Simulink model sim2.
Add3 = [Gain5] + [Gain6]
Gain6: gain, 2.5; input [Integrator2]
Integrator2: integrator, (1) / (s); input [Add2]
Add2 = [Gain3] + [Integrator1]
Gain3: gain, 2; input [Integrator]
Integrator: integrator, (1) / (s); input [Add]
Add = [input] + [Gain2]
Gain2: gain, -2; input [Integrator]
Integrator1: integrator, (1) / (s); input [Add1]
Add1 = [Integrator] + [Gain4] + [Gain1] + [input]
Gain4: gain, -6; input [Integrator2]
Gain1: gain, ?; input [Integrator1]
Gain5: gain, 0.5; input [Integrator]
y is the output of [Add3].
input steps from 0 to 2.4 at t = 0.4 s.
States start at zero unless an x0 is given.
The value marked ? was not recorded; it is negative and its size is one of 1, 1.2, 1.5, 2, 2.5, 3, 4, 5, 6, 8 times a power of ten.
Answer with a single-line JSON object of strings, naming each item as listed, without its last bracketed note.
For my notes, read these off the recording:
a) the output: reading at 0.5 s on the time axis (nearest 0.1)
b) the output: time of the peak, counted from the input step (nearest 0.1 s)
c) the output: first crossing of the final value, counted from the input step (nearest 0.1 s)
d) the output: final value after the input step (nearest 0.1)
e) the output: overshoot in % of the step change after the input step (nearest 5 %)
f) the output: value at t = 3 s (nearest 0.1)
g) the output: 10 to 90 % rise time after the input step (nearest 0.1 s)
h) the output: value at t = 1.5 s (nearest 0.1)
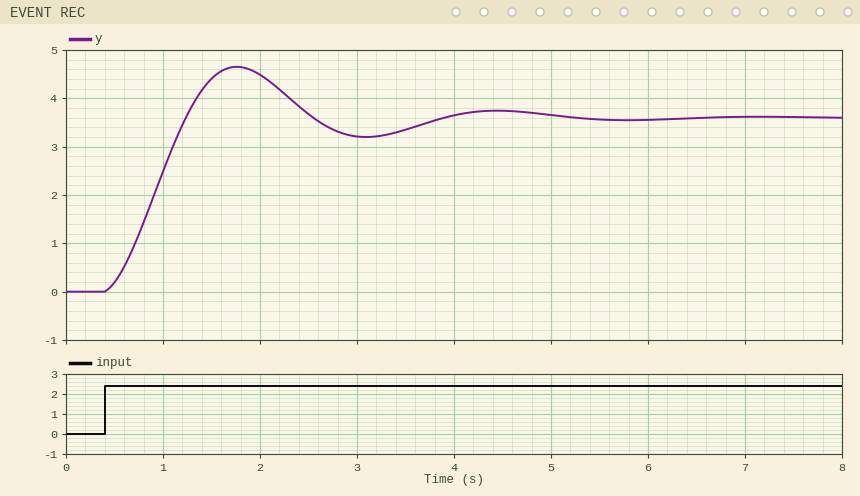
{"the output: reading at 0.5 s on the time axis": "0.2", "the output: time of the peak, counted from the input step": "1.4 s", "the output: first crossing of the final value, counted from the input step": "0.8 s", "the output: final value after the input step": "3.6", "the output: overshoot in % of the step change after the input step": "30 %", "the output: value at t = 3 s": "3.2", "the output: 10 to 90 % rise time after the input step": "0.6 s", "the output: value at t = 1.5 s": "4.4"}
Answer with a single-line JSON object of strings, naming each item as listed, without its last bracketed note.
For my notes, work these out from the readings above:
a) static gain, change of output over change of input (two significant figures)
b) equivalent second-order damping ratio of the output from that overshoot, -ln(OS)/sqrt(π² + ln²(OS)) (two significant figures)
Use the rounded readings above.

{"static gain, change of output over change of input": "1.5", "equivalent second-order damping ratio of the output from that overshoot, -ln(OS)/sqrt(π² + ln²(OS))": "0.36"}
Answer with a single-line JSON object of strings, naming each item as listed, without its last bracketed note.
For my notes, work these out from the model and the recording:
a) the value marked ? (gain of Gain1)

{"the value marked ?": "-1.5"}
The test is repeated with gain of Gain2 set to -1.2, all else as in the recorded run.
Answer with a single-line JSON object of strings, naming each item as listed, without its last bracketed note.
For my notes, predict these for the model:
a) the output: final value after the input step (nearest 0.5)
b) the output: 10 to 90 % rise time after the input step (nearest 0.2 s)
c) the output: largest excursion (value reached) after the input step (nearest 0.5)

{"the output: final value after the input step": "5.5", "the output: 10 to 90 % rise time after the input step": "0.8 s", "the output: largest excursion (value reached) after the input step": "6.0"}
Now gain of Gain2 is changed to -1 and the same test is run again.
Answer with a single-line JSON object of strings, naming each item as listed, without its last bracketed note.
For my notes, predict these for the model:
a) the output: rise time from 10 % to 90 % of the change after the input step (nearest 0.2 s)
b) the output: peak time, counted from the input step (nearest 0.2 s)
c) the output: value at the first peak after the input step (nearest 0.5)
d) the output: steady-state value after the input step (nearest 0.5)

{"the output: rise time from 10 % to 90 % of the change after the input step": "0.8 s", "the output: peak time, counted from the input step": "1.6 s", "the output: value at the first peak after the input step": "6.5", "the output: steady-state value after the input step": "6.0"}
